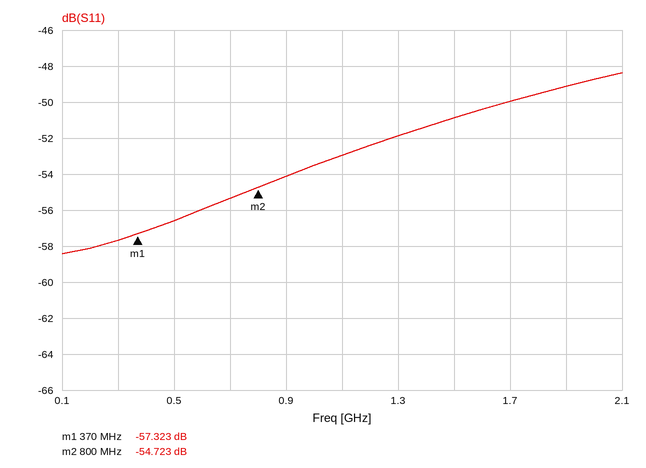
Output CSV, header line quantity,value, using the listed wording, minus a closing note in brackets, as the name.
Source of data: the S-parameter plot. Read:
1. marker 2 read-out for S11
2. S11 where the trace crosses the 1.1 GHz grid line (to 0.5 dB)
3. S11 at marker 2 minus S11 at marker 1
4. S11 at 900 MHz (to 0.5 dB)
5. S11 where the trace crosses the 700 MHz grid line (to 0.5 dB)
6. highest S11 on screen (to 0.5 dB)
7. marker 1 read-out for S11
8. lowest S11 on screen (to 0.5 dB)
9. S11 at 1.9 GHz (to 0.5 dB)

quantity,value
marker 2 read-out for S11,-54.723 dB
S11 where the trace crosses the 1.1 GHz grid line,-53.0 dB
S11 at marker 2 minus S11 at marker 1,2.600 dB
S11 at 900 MHz,-54.0 dB
S11 where the trace crosses the 700 MHz grid line,-55.5 dB
highest S11 on screen,-48.5 dB
marker 1 read-out for S11,-57.323 dB
lowest S11 on screen,-58.5 dB
S11 at 1.9 GHz,-49.0 dB
